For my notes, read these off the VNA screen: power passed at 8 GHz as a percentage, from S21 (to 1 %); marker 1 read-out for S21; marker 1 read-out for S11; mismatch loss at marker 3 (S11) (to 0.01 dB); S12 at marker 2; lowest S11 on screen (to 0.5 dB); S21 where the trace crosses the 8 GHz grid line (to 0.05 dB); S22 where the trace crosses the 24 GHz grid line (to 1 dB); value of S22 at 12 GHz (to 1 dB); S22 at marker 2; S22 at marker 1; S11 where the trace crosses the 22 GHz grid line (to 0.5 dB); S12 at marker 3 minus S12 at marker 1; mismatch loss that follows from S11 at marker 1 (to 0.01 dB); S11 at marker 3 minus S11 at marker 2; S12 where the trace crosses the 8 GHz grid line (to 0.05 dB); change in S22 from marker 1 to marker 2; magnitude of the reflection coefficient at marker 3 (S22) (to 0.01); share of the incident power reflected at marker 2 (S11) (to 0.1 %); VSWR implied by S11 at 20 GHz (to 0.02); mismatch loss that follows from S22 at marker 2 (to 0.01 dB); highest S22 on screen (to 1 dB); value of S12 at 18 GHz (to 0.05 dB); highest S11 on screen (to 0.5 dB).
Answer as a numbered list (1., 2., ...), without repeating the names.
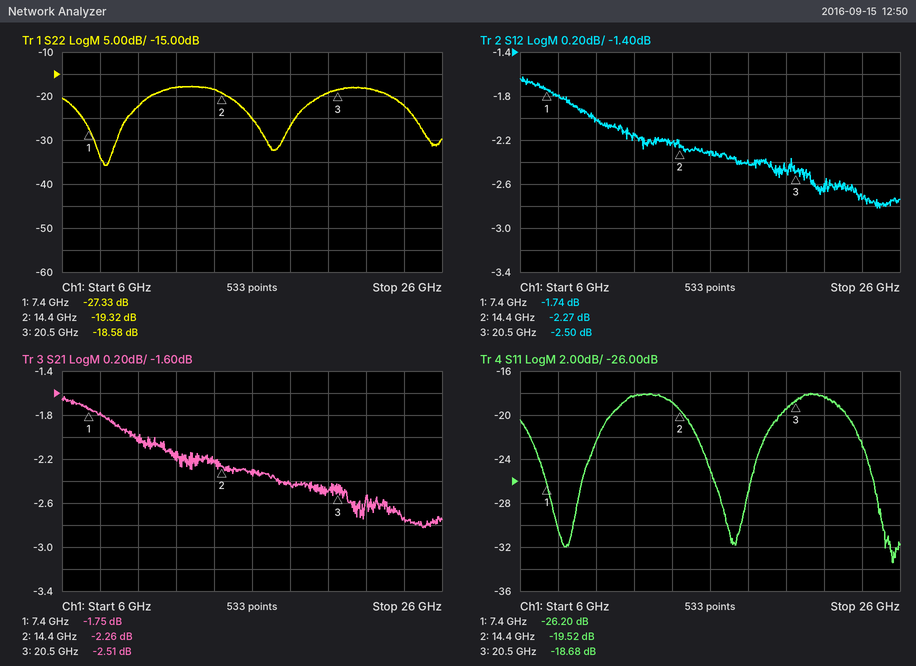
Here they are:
1. 66 %
2. -1.75 dB
3. -26.20 dB
4. 0.06 dB
5. -2.27 dB
6. -33.5 dB
7. -1.80 dB
8. -22 dB
9. -18 dB
10. -19.32 dB
11. -27.33 dB
12. -18.5 dB
13. -0.76 dB
14. 0.01 dB
15. 0.84 dB
16. -1.80 dB
17. 8.01 dB
18. 0.12
19. 1.1 %
20. 1.24
21. 0.05 dB
22. -18 dB
23. -2.40 dB
24. -18.0 dB
